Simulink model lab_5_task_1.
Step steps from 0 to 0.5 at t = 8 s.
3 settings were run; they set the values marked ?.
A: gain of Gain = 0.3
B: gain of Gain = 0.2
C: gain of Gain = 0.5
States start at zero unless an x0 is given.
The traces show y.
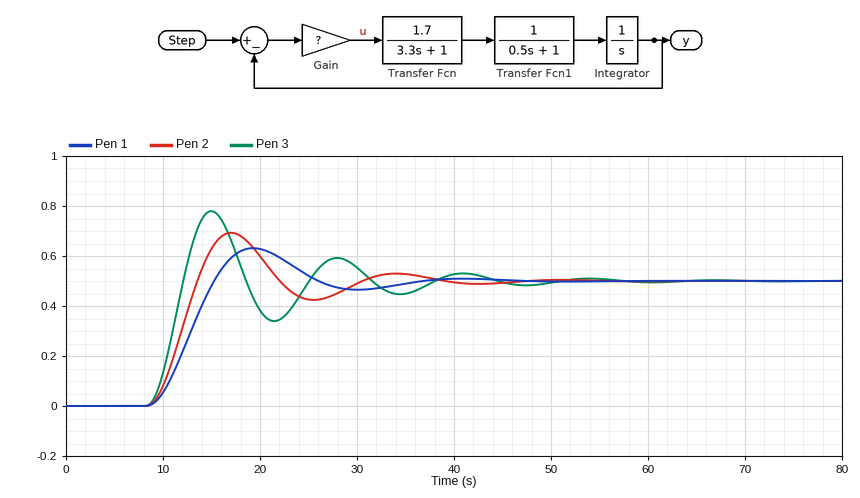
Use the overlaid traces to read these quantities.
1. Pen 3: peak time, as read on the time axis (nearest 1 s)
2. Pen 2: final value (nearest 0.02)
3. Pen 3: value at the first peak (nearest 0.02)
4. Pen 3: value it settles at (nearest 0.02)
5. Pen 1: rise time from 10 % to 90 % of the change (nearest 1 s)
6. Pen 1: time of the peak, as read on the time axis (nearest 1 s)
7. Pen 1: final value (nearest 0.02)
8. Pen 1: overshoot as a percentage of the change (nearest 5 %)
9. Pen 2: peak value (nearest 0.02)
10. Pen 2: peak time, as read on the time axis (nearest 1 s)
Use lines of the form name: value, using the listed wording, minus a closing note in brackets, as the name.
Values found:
Pen 3: peak time, as read on the time axis: 15 s
Pen 2: final value: 0.50
Pen 3: value at the first peak: 0.78
Pen 3: value it settles at: 0.50
Pen 1: rise time from 10 % to 90 % of the change: 5 s
Pen 1: time of the peak, as read on the time axis: 19 s
Pen 1: final value: 0.50
Pen 1: overshoot as a percentage of the change: 25 %
Pen 2: peak value: 0.70
Pen 2: peak time, as read on the time axis: 17 s
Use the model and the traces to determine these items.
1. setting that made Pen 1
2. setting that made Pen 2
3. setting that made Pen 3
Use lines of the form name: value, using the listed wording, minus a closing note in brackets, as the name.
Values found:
setting that made Pen 1: B
setting that made Pen 2: A
setting that made Pen 3: C
